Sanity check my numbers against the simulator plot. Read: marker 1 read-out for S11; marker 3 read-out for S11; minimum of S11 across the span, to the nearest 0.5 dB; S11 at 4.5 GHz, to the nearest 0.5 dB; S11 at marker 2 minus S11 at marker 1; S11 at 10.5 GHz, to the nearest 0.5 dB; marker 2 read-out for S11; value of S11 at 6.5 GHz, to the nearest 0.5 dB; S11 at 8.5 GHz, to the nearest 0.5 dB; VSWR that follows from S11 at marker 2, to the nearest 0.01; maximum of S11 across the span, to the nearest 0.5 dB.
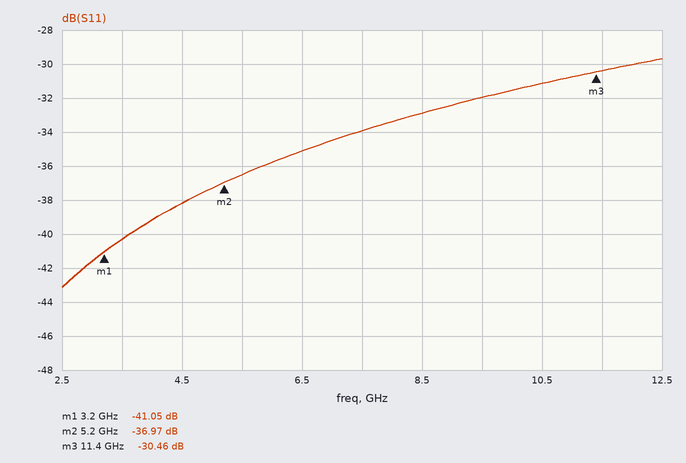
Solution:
-41.05 dB
-30.46 dB
-43.0 dB
-38.0 dB
4.08 dB
-31.0 dB
-36.97 dB
-35.0 dB
-33.0 dB
1.03
-29.5 dB
